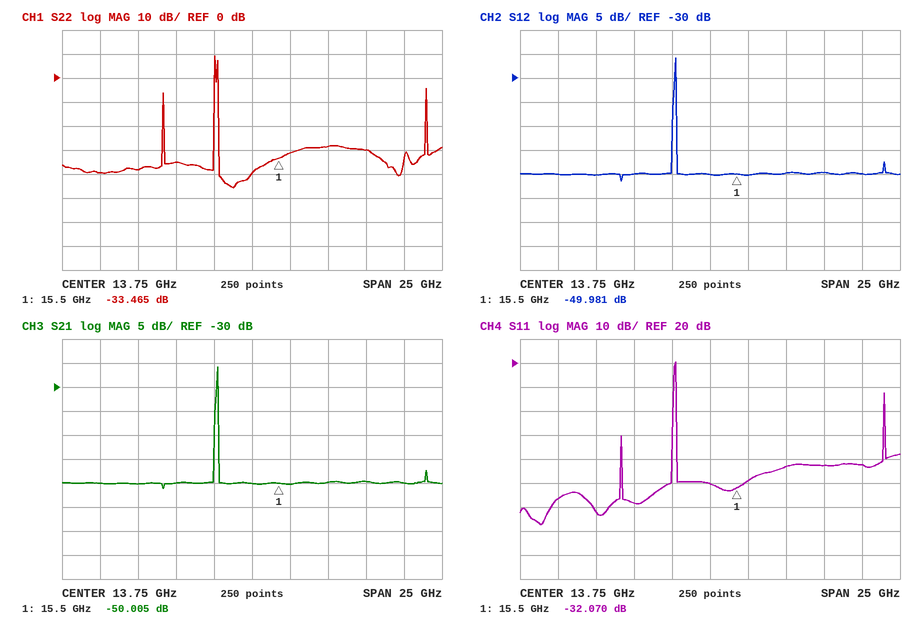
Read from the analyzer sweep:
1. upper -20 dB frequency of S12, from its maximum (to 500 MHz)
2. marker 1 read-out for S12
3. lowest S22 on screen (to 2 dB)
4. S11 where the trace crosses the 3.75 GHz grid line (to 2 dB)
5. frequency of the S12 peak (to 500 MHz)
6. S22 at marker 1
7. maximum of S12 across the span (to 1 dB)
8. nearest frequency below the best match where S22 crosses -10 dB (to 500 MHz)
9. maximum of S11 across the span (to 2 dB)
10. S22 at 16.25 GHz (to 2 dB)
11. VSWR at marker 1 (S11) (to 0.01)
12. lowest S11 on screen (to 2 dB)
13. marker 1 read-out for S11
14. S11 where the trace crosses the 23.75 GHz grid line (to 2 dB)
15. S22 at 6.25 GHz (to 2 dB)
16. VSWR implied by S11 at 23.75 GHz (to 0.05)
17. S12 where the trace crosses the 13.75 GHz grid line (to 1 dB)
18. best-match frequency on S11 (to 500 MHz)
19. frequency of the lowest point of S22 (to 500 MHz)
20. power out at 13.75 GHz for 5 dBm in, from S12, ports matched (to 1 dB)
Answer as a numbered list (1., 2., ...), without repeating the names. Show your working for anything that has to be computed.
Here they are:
1. 11.5 GHz
2. -49.981 dB
3. -46 dB
4. -36 dB
5. 11.5 GHz
6. -33.465 dB
7. -26 dB
8. 11.5 GHz
9. 20 dB
10. -32 dB
11. (1 + 0.0249)/(1 − 0.0249) ≈ 1.05
12. -48 dB
13. -32.070 dB
14. -22 dB
15. -38 dB
16. |Γ| = 10^(-22/20) = 0.0794; VSWR = (1 + 0.0794)/(1 − 0.0794) ≈ 1.17, so 1.15 to the nearest 0.05
17. -50 dB
18. 2.5 GHz
19. 12.5 GHz
20. 5 dBm + (-50 dB) = -45 dBm
